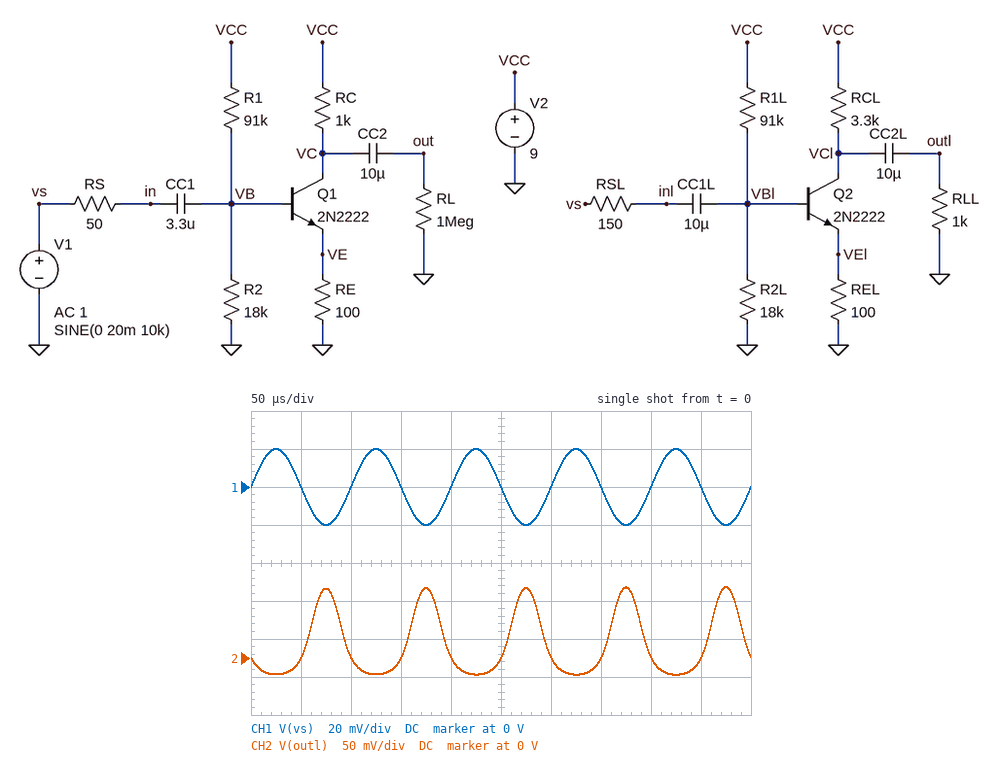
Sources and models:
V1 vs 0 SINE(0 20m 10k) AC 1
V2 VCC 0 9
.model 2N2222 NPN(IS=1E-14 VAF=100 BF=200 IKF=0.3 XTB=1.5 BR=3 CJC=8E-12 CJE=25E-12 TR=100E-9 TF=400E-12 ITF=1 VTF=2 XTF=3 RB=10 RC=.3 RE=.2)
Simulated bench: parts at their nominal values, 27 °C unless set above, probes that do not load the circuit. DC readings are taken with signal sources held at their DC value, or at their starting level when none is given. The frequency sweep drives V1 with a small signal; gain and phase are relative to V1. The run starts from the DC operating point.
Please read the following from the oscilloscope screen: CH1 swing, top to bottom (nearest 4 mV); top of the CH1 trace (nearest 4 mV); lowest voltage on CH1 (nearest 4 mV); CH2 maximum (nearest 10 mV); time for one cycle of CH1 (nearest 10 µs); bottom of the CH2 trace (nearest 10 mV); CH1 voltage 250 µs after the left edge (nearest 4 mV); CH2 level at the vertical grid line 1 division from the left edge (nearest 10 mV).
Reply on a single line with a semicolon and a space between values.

40 mV; 20 mV; -20 mV; 90 mV; 100 µs; -20 mV; 0 V; 0 V
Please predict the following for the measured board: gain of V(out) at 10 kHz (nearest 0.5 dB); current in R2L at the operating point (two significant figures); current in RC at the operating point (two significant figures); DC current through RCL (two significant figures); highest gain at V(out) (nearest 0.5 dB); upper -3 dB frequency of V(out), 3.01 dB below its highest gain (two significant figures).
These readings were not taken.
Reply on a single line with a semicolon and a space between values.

19.5 dB; 53 µA; 4.5 mA; 2.6 mA; 19.5 dB; 21 MHz
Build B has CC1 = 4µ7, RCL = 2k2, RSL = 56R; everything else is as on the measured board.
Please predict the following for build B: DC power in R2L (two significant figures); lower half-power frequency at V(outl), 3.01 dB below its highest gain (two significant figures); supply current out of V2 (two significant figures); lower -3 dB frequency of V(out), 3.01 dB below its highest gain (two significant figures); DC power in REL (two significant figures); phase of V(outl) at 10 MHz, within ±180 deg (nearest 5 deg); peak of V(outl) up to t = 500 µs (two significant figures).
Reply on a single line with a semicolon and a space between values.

65 µW; 25 Hz; 8.6 mA; 3.9 Hz; 1.5 mW; 65 deg; 120 mV
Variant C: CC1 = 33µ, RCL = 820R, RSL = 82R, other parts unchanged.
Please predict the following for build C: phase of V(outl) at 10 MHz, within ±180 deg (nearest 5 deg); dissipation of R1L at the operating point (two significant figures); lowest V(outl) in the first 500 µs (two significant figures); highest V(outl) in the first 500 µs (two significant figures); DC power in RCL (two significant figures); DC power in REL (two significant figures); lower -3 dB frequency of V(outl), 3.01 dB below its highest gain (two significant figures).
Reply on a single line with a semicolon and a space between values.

160 deg; 680 µW; -84 mV; 84 mV; 17 mW; 2.1 mW; 9.1 Hz
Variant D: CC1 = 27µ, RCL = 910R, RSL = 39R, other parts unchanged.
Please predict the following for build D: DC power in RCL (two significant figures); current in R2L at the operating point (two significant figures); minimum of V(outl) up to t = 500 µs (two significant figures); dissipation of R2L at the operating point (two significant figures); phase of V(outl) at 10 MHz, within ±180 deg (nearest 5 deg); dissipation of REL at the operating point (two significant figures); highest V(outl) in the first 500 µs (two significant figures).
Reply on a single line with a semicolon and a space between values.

19 mW; 64 µA; -89 mV; 74 µW; 165 deg; 2.1 mW; 89 mV
